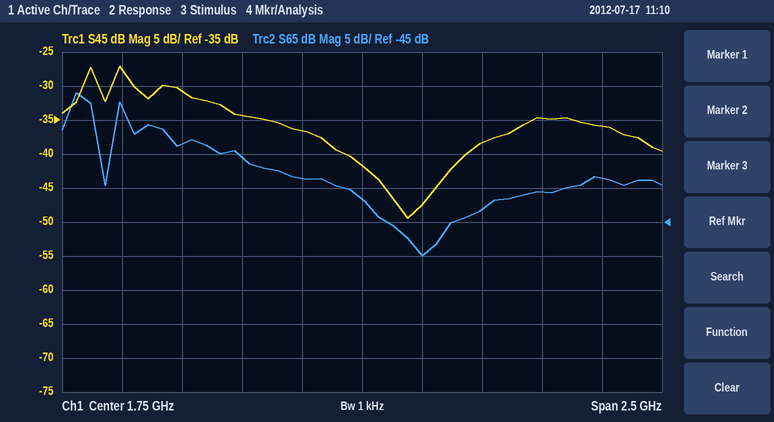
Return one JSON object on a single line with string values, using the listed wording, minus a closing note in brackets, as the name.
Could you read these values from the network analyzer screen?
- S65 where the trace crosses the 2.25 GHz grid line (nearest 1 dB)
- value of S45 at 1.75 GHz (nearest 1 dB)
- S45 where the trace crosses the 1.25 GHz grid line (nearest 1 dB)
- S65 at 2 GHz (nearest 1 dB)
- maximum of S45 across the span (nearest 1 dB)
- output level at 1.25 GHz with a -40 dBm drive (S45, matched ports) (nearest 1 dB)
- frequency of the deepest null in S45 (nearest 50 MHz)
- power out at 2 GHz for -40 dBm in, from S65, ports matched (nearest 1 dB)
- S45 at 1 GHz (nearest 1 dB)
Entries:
{"S65 where the trace crosses the 2.25 GHz grid line": "-43 dB", "value of S45 at 1.75 GHz": "-42 dB", "S45 where the trace crosses the 1.25 GHz grid line": "-34 dB", "S65 at 2 GHz": "-50 dB", "maximum of S45 across the span": "-27 dB", "output level at 1.25 GHz with a -40 dBm drive (S45, matched ports)": "-74 dBm", "frequency of the deepest null in S45": "1.95 GHz", "power out at 2 GHz for -40 dBm in, from S65, ports matched": "-90 dBm", "S45 at 1 GHz": "-31 dB"}
